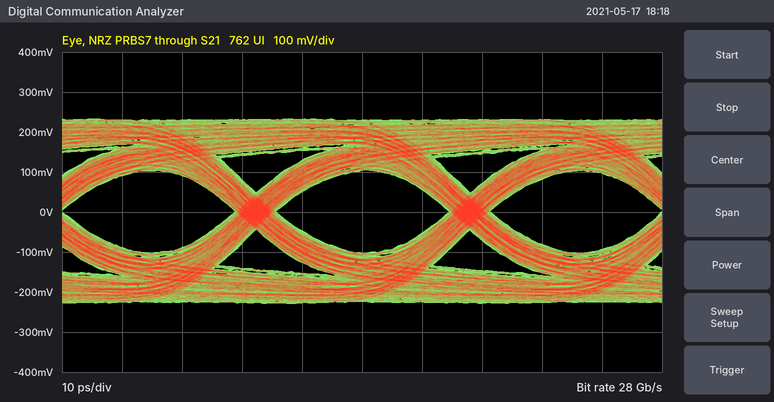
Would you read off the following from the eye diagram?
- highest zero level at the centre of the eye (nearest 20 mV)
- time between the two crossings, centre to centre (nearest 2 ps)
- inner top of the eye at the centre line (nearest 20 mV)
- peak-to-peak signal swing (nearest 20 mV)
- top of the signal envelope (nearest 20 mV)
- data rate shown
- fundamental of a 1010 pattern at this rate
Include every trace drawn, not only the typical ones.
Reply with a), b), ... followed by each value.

a) -100 mV
b) 36 ps
c) 100 mV
d) 460 mV
e) 240 mV
f) 28 Gb/s
g) 14 GHz
